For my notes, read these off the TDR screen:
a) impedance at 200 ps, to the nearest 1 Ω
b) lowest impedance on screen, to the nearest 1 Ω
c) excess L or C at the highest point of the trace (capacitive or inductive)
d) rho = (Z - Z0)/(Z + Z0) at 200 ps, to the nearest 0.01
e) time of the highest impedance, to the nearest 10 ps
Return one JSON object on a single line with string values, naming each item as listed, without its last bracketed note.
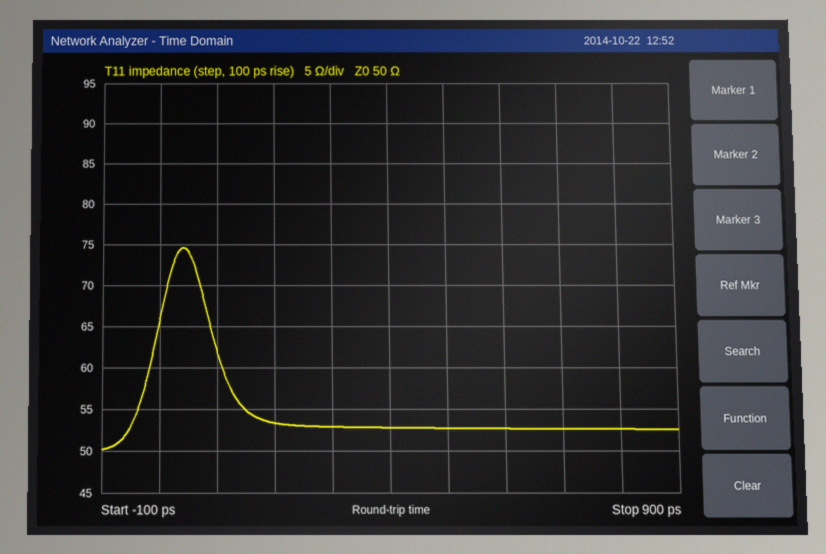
{"impedance at 200 ps, to the nearest 1 Ω": "53 Ω", "lowest impedance on screen, to the nearest 1 Ω": "50 Ω", "excess L or C at the highest point of the trace": "inductive", "rho = (Z - Z0)/(Z + Z0) at 200 ps, to the nearest 0.01": "+0.03", "time of the highest impedance, to the nearest 10 ps": "40 ps"}
